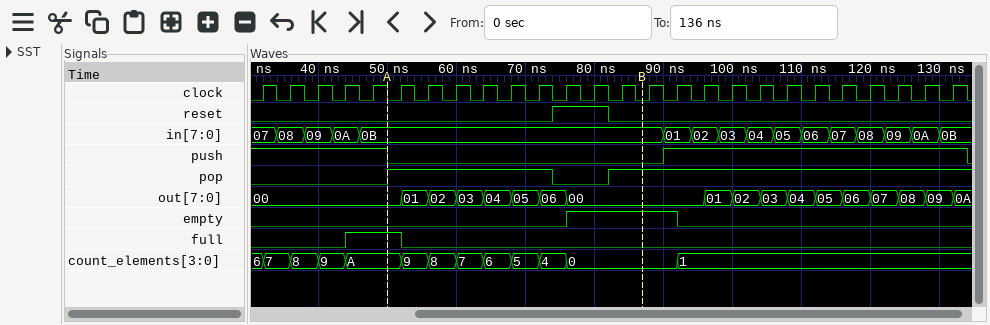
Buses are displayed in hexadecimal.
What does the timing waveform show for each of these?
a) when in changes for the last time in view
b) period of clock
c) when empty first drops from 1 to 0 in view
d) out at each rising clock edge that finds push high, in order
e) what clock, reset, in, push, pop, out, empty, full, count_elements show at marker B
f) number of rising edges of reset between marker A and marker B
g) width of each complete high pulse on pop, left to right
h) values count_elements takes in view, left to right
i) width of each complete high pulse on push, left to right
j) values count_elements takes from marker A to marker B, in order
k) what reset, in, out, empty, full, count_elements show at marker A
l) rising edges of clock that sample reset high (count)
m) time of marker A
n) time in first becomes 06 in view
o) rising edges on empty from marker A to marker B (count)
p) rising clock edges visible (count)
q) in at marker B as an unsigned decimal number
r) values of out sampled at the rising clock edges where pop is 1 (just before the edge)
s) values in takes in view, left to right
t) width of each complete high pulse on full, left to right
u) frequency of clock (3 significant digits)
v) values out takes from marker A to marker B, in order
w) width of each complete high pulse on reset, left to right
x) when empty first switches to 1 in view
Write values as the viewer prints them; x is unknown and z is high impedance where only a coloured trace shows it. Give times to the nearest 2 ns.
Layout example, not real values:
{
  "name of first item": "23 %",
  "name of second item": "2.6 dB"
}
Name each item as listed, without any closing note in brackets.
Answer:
{
  "when in changes for the last time in view": "130 ns",
  "period of clock": "4 ns",
  "when empty first drops from 1 to 0 in view": "92 ns",
  "out at each rising clock edge that finds push high, in order": "00, 00, 00, 00, 00, 00, 00, 01, 02, 03, 04, 05, 06, 07, 08, 09",
  "what clock, reset, in, push, pop, out, empty, full, count_elements show at marker B": "clock=0, reset=0, in=0B, push=0, pop=1, out=00, empty=1, full=0, count_elements=0",
  "number of rising edges of reset between marker A and marker B": "1",
  "width of each complete high pulse on pop, left to right": "24 ns",
  "values count_elements takes in view, left to right": "6, 7, 8, 9, A, 9, 8, 7, 6, 5, 4, 0, 1",
  "width of each complete high pulse on push, left to right": "44 ns",
  "values count_elements takes from marker A to marker B, in order": "A, 9, 8, 7, 6, 5, 4, 0",
  "what reset, in, out, empty, full, count_elements show at marker A": "reset=0, in=0B, out=00, empty=0, full=1, count_elements=A",
  "rising edges of clock that sample reset high": "2",
  "time of marker A": "50 ns",
  "time in first becomes 06 in view": "110 ns",
  "rising edges on empty from marker A to marker B": "1",
  "rising clock edges visible": "26",
  "in at marker B as an unsigned decimal number": "11",
  "values of out sampled at the rising clock edges where pop is 1": "00, 01, 02, 03, 04, 05, 00, 00, 00, 00, 01, 02, 03, 04, 05, 06, 07, 08, 09",
  "values in takes in view, left to right": "07, 08, 09, 0A, 0B, 01, 02, 03, 04, 05, 06, 07, 08, 09, 0A, 0B",
  "width of each complete high pulse on full, left to right": "8 ns",
  "frequency of clock": "250 MHz",
  "values out takes from marker A to marker B, in order": "00, 01, 02, 03, 04, 05, 06, 00",
  "width of each complete high pulse on reset, left to right": "8 ns",
  "when empty first switches to 1 in view": "76 ns"
}
